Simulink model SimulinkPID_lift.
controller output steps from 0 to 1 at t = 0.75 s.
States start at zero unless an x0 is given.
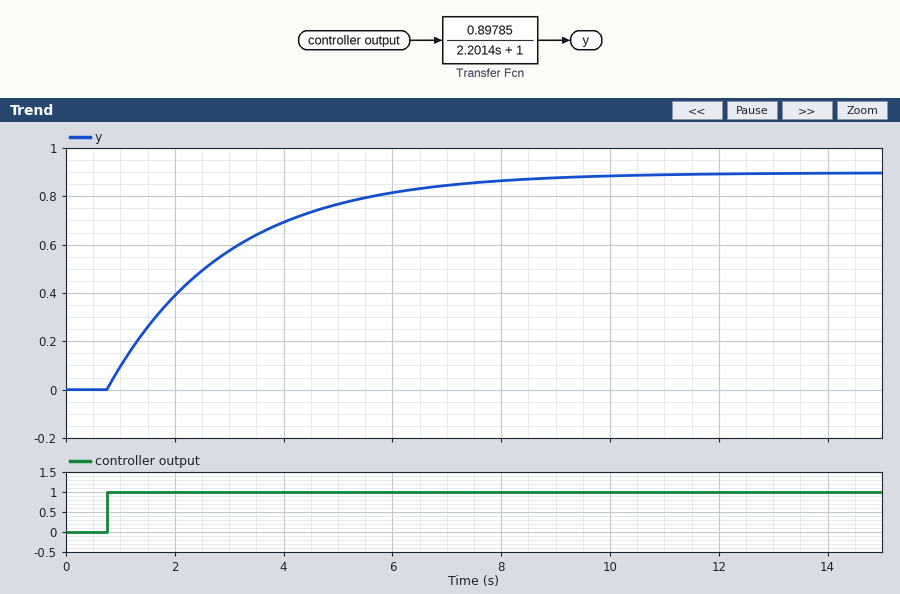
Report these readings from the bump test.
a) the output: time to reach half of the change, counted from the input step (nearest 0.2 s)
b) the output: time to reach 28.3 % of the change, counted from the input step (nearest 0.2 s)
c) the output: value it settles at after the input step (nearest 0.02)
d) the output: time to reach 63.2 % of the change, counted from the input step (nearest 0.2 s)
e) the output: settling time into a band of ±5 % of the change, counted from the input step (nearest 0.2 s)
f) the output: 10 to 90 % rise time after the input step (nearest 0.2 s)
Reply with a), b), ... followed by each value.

a) 1.6 s
b) 0.8 s
c) 0.90
d) 2.2 s
e) 6.6 s
f) 4.8 s
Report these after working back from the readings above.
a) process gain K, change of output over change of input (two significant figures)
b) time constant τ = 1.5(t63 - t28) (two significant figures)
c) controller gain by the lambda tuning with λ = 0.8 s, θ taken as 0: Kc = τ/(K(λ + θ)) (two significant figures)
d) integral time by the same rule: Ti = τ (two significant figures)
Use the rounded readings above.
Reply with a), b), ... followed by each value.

a) 0.90
b) 2.1 s
c) 2.9
d) 2.1 s
